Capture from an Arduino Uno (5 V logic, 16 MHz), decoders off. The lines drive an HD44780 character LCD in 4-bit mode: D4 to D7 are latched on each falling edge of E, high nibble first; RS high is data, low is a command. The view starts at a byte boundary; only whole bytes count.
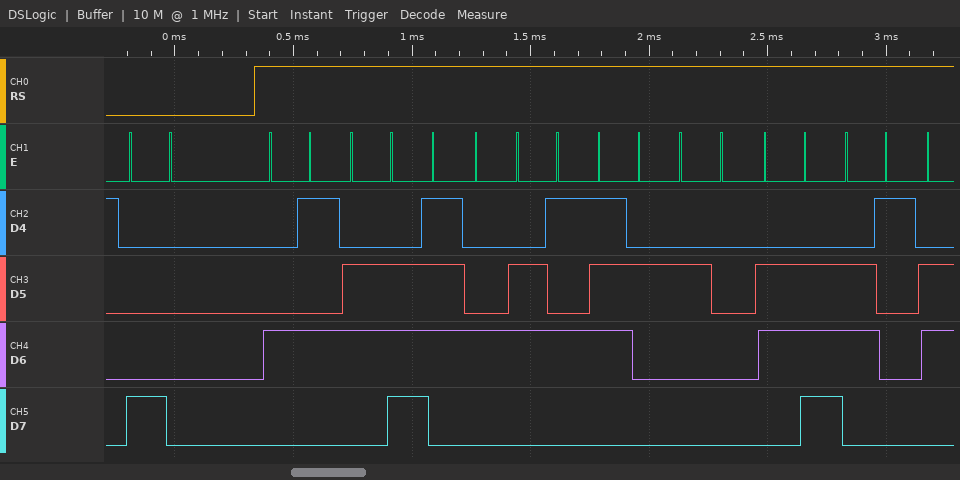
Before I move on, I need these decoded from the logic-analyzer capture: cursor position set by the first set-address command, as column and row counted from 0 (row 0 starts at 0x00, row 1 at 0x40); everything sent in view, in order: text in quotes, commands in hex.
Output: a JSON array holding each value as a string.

["column 0, row 0", "0x80 \"Enter na\""]
